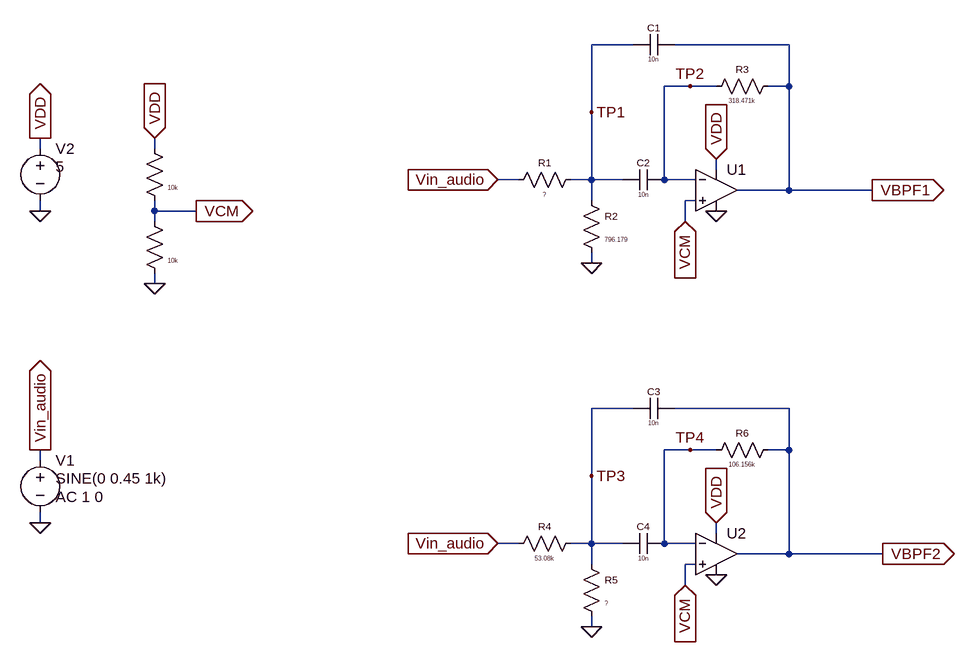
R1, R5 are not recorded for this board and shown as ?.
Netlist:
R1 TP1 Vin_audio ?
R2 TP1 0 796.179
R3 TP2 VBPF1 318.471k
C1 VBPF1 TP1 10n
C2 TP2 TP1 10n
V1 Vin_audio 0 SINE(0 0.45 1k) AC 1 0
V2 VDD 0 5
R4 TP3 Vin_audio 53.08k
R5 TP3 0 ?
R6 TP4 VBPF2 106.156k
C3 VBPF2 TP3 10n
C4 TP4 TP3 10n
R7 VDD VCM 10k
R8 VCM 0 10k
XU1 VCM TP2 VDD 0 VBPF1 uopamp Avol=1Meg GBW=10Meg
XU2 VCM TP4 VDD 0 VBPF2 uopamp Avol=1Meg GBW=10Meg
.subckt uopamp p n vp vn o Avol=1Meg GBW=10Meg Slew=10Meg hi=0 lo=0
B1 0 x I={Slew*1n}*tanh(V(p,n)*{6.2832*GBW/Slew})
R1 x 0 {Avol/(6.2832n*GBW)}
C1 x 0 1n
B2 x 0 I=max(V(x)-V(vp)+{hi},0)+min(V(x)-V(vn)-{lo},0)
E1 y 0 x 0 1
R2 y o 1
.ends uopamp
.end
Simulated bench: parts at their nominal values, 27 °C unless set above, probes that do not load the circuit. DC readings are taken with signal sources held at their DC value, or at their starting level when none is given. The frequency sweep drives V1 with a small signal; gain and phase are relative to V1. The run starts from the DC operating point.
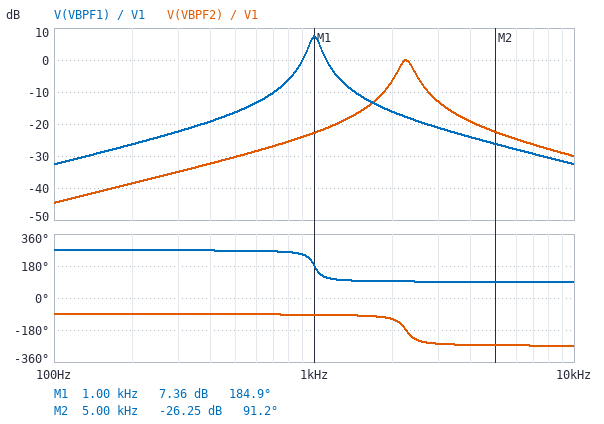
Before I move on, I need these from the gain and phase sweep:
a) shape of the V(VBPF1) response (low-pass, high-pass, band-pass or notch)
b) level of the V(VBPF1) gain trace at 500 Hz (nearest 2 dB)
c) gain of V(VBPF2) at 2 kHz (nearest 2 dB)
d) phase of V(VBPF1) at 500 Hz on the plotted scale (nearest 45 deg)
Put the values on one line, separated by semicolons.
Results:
band-pass; -16 dB; -6 dB; 270 deg
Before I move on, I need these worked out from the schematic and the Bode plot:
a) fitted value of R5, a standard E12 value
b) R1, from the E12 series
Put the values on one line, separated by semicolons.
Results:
470 Ω; 68 kΩ
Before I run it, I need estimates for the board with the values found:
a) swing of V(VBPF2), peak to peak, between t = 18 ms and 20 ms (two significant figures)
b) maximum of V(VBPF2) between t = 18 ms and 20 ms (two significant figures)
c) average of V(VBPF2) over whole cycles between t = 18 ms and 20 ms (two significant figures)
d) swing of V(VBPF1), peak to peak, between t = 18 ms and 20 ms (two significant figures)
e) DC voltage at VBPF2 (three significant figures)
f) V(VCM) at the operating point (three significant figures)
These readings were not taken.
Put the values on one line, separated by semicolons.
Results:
65 mV; 2.5 V; 2.5 V; 2.1 V; 2.50 V; 2.50 V
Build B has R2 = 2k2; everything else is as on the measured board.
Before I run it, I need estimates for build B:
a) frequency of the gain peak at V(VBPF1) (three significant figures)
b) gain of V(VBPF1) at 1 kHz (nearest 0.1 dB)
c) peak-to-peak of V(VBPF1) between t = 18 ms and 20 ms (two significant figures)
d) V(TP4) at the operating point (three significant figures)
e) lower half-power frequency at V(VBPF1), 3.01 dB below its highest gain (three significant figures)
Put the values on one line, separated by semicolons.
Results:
611 Hz; -8.7 dB; 330 mV; 2.50 V; 563 Hz
